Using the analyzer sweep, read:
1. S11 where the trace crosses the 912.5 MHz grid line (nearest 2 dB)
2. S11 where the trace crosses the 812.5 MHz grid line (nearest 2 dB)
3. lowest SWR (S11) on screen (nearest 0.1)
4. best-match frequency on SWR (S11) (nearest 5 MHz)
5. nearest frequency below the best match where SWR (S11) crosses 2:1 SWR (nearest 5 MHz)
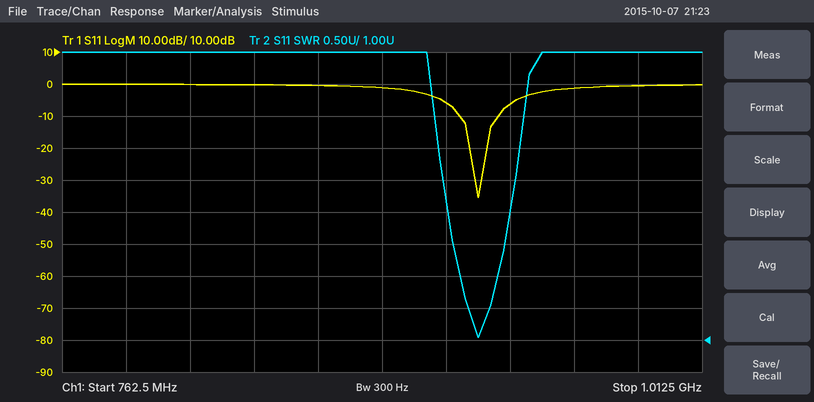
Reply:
-6 dB
0 dB
1.0
925 MHz
920 MHz
